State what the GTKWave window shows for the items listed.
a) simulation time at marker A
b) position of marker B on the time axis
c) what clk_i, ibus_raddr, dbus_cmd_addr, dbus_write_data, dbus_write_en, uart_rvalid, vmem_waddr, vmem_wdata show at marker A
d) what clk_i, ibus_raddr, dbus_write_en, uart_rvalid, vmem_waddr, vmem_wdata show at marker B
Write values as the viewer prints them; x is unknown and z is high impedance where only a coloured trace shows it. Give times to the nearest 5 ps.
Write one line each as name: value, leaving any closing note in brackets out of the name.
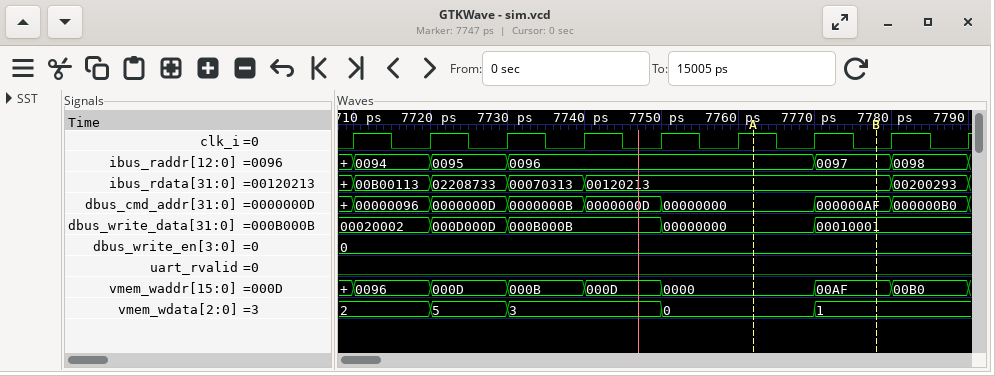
simulation time at marker A: 7760 ps
position of marker B on the time axis: 7780 ps
what clk_i, ibus_raddr, dbus_cmd_addr, dbus_write_data, dbus_write_en, uart_rvalid, vmem_waddr, vmem_wdata show at marker A: clk_i=1, ibus_raddr=0096, dbus_cmd_addr=00000000, dbus_write_data=00000000, dbus_write_en=0, uart_rvalid=0, vmem_waddr=0000, vmem_wdata=0
what clk_i, ibus_raddr, dbus_write_en, uart_rvalid, vmem_waddr, vmem_wdata show at marker B: clk_i=0, ibus_raddr=0097, dbus_write_en=0, uart_rvalid=0, vmem_waddr=00AF, vmem_wdata=1
